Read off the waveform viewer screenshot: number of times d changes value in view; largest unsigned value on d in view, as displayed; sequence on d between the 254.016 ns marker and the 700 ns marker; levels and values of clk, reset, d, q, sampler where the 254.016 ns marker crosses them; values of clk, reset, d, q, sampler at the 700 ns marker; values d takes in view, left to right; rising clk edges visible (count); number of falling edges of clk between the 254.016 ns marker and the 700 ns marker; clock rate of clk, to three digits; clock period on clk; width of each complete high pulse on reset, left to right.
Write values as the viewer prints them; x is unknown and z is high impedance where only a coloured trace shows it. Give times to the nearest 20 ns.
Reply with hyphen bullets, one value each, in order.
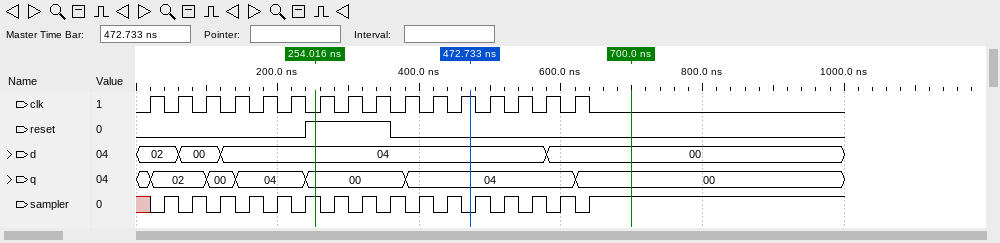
- 3
- 04
- 04, 00
- clk=0, reset=1, d=04, q=00, sampler=1
- clk=0, reset=0, d=00, q=00, sampler=1
- 02, 00, 04, 00
- 16
- 10
- 25.0 MHz
- 40 ns
- 120 ns
